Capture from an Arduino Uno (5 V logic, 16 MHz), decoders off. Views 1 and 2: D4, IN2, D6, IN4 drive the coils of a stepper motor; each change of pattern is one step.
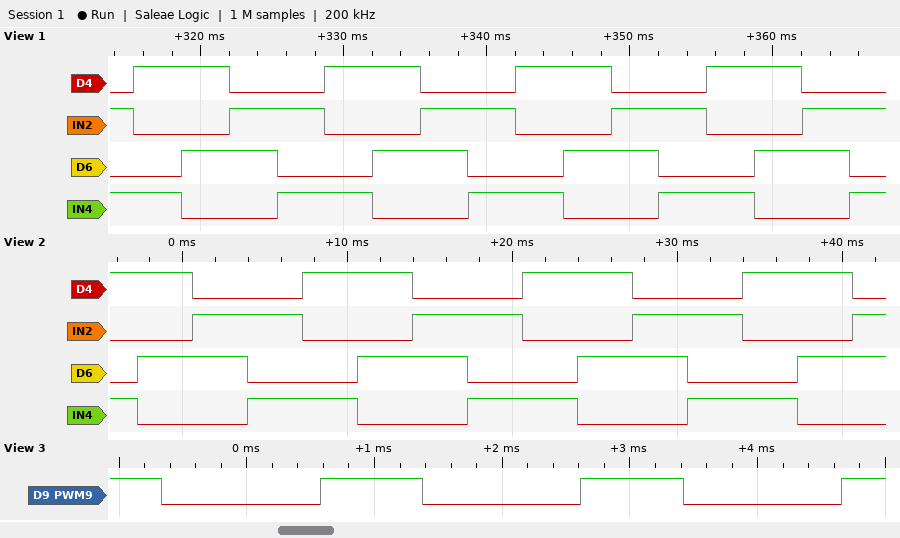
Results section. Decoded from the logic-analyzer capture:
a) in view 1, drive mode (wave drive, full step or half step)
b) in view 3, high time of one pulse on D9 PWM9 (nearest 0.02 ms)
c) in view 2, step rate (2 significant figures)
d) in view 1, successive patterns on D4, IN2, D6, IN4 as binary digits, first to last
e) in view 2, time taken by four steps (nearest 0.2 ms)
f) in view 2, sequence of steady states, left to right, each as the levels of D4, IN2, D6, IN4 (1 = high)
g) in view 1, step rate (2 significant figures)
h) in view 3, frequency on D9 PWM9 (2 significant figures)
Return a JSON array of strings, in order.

["full step", "0.80 ms", "300 steps/s", "0101 1001 1010 0110 0101 1001 1010 0110 0101 1001 1010 0110 0101 1001 1010 0110 0101", "13.4 ms", "1001 1010 0110 0101 1001 1010 0110 0101 1001 1010 0110 0101 1001 1010 0110", "300 steps/s", "490 Hz"]
